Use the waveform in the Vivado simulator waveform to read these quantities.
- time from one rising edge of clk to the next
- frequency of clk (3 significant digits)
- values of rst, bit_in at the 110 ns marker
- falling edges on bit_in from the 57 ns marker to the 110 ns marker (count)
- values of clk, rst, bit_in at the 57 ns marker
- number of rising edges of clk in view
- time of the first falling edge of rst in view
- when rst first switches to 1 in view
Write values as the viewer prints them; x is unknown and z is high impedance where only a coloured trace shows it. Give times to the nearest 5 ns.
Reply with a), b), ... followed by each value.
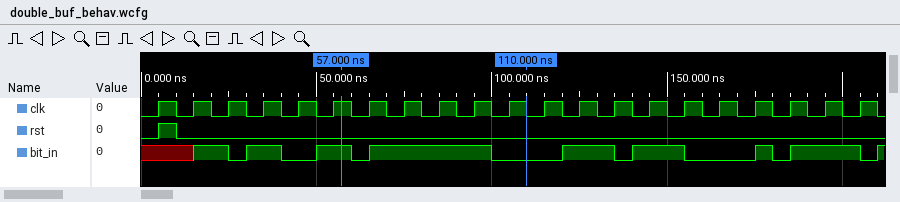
a) 10 ns
b) 100 MHz
c) rst=0, bit_in=0
d) 2
e) clk=1, rst=0, bit_in=1
f) 21
g) 10 ns
h) 5 ns
